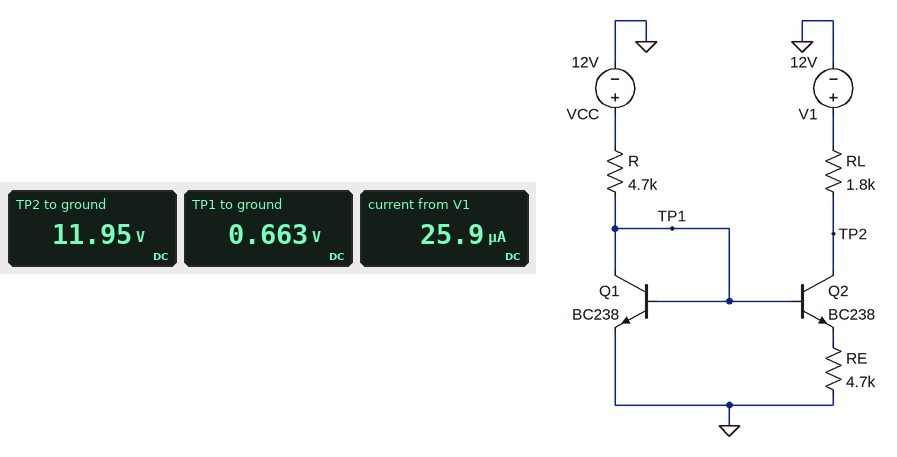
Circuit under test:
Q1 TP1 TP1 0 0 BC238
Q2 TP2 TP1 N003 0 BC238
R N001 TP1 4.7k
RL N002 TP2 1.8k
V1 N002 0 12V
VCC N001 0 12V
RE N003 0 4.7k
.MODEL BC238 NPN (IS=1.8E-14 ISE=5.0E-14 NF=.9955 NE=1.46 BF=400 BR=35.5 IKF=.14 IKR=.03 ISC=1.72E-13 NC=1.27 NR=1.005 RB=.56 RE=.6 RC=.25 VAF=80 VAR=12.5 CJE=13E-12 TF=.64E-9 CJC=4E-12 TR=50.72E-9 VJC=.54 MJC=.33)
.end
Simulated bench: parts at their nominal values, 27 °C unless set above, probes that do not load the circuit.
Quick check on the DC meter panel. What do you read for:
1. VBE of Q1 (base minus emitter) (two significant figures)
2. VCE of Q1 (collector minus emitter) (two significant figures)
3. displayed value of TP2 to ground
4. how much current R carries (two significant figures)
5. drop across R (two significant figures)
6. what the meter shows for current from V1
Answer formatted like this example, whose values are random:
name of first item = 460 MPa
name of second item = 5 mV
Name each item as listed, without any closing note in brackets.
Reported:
VBE of Q1 (base minus emitter) = 660 mV
VCE of Q1 (collector minus emitter) = 660 mV
displayed value of TP2 to ground = 11.95 V
how much current R carries = 2.4 mA
drop across R = 11 V
what the meter shows for current from V1 = 25.9 µA
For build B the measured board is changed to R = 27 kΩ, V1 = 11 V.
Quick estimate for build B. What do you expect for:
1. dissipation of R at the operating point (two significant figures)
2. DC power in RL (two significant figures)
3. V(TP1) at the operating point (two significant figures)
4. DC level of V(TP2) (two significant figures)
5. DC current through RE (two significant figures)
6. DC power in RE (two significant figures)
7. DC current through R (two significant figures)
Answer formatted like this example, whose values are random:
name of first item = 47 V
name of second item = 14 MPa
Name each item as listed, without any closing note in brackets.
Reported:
dissipation of R at the operating point = 4.8 mW
DC power in RL = 580 nW
V(TP1) at the operating point = 620 mV
DC level of V(TP2) = 11 V
DC current through RE = 18 µA
DC power in RE = 1.5 µW
DC current through R = 420 µA
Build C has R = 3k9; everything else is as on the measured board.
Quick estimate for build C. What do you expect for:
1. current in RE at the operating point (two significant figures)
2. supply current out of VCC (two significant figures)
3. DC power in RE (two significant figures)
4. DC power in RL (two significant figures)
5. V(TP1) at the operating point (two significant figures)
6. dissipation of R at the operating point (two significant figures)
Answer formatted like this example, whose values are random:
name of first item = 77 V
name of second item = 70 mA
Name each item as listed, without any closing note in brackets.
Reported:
current in RE at the operating point = 27 µA
supply current out of VCC = 2.9 mA
DC power in RE = 3.4 µW
DC power in RL = 1.3 µW
V(TP1) at the operating point = 670 mV
dissipation of R at the operating point = 33 mW
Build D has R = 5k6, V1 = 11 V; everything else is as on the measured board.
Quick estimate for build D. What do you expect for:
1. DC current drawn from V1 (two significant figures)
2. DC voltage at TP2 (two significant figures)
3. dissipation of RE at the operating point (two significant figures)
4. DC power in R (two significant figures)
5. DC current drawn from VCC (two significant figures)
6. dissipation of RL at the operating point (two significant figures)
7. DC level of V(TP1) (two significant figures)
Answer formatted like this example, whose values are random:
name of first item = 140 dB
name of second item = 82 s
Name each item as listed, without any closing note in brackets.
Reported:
DC current drawn from V1 = 25 µA
DC voltage at TP2 = 11 V
dissipation of RE at the operating point = 3.0 µW
DC power in R = 23 mW
DC current drawn from VCC = 2.0 mA
dissipation of RL at the operating point = 1.1 µW
DC level of V(TP1) = 660 mV
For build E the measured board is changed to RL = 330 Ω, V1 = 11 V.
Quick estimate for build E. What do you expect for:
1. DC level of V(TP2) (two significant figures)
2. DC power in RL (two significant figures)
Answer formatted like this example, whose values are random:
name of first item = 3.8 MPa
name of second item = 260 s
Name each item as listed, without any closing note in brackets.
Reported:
DC level of V(TP2) = 11 V
DC power in RL = 220 nW
